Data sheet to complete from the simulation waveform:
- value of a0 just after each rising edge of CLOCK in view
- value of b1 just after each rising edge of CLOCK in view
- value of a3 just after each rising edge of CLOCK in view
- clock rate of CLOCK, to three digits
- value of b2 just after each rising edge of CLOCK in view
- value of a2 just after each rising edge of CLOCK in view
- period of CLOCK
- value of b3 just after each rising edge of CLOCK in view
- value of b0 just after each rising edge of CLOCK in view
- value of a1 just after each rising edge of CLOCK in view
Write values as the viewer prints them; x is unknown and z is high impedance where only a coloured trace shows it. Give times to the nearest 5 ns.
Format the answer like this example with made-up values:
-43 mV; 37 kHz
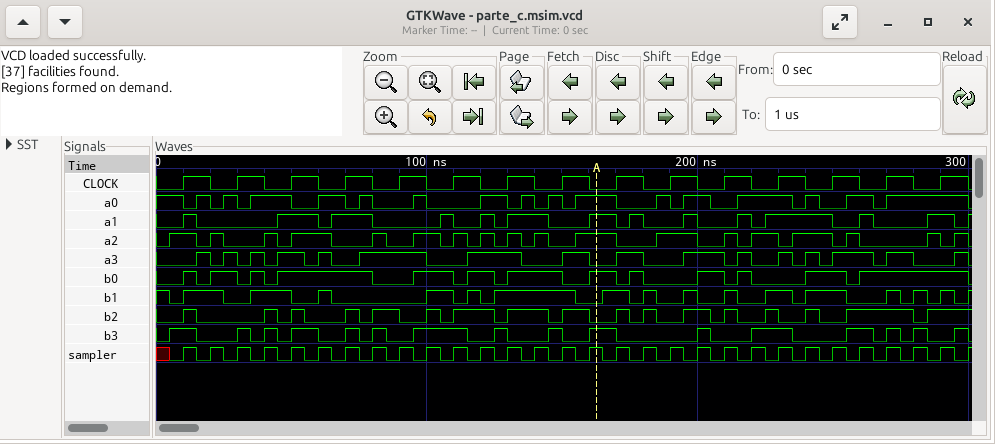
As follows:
0 0 0 0 0 0 0 0 0 0 0 1 0 1 1; 1 0 0 0 0 0 1 1 1 0 1 1 1 1 1; 0 0 1 0 1 0 1 1 1 0 0 1 1 1 0; 50.0 MHz; 1 0 1 1 0 1 1 1 1 0 1 0 0 1 1; 1 0 1 0 0 1 1 0 0 1 1 0 0 0 0; 20 ns; 1 1 1 1 0 1 0 0 0 0 0 1 0 1 0; 1 0 1 1 0 0 1 0 0 0 0 0 1 1 1; 1 0 1 1 0 0 1 0 0 0 0 1 0 0 1
